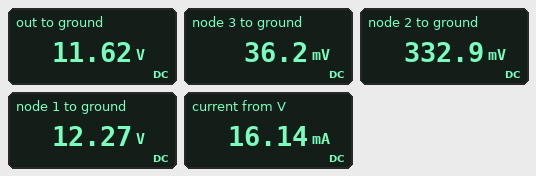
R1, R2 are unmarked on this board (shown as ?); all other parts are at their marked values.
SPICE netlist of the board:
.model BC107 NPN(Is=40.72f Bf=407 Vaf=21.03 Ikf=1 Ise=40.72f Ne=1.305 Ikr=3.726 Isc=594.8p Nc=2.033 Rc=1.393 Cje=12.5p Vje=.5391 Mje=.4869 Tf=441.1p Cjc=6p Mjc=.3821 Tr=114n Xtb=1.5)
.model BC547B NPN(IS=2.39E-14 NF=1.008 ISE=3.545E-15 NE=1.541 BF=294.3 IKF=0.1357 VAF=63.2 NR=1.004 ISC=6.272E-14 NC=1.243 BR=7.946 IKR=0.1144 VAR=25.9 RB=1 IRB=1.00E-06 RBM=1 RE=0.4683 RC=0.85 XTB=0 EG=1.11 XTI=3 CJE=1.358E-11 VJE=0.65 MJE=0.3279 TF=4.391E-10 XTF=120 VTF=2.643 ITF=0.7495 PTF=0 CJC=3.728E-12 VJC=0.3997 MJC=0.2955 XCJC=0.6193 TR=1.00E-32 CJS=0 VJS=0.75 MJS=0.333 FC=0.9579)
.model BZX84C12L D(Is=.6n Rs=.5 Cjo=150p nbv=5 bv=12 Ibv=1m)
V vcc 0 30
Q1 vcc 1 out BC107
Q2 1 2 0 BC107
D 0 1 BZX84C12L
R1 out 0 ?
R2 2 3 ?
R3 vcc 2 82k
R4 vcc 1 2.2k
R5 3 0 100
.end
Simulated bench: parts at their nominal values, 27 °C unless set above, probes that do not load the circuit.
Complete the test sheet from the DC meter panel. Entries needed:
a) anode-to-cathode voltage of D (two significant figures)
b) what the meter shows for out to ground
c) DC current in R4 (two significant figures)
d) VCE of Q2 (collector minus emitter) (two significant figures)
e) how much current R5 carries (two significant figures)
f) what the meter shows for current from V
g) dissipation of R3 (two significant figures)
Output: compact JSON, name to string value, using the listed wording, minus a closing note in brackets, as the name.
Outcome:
{"anode-to-cathode voltage of D": "-12 V", "what the meter shows for out to ground": "11.62 V", "DC current in R4": "8.1 mA", "VCE of Q2 (collector minus emitter)": "12 V", "how much current R5 carries": "360 µA", "what the meter shows for current from V": "16.14 mA", "dissipation of R3": "11 mW"}
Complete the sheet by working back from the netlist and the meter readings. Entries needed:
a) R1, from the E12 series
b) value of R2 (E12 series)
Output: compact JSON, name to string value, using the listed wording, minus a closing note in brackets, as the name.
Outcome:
{"R1, from the E12 series": "1.5 kΩ", "value of R2": "820 Ω"}
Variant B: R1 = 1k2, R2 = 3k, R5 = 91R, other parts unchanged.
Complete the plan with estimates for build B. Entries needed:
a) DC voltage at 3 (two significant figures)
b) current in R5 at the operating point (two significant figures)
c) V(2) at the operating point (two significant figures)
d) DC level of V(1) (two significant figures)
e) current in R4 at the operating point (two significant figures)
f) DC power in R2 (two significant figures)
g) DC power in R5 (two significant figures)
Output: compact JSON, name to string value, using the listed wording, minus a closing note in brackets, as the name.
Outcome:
{"DC voltage at 3": "20 mV", "current in R5 at the operating point": "220 µA", "V(2) at the operating point": "690 mV", "DC level of V(1)": "160 mV", "current in R4 at the operating point": "14 mA", "DC power in R2": "150 µW", "DC power in R5": "4.5 µW"}
